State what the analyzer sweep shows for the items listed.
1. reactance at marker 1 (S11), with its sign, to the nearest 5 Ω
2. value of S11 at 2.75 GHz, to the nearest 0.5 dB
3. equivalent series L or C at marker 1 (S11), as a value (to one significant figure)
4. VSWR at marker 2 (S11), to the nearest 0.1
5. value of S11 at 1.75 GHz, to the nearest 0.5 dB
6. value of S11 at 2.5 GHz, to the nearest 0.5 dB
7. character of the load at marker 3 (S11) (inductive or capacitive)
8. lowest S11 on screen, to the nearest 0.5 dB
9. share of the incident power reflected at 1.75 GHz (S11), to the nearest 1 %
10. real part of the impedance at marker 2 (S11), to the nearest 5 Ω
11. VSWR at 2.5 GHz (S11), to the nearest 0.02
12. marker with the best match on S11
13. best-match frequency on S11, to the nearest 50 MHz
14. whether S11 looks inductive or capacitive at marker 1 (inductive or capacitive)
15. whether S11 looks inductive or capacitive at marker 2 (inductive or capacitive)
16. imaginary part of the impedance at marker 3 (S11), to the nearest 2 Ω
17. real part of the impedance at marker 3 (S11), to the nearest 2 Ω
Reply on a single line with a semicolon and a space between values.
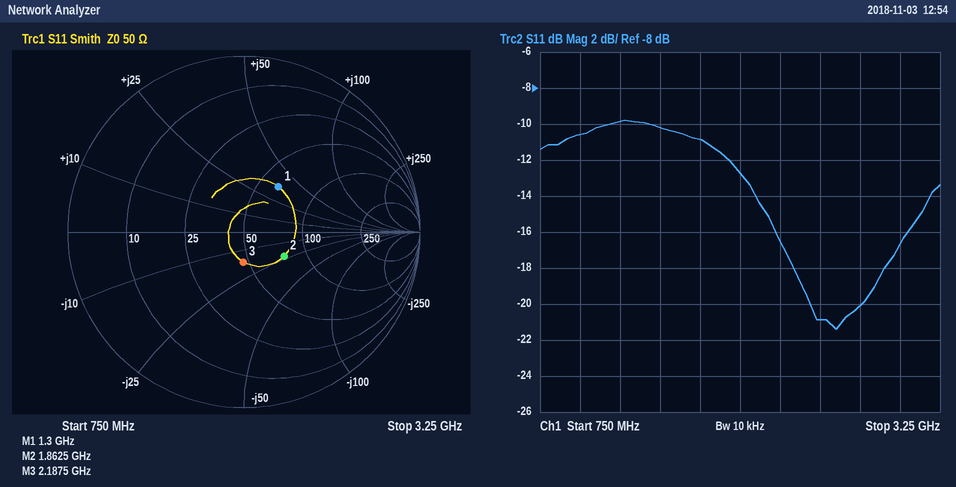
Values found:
+35 Ω; -20.0 dB; 4 nH; 1.7; -11.0 dB; -21.0 dB; capacitive; -21.5 dB; 8 %; 75 Ω; 1.20; marker 3; 2.60 GHz; inductive; capacitive; -16 Ω; 46 Ω
